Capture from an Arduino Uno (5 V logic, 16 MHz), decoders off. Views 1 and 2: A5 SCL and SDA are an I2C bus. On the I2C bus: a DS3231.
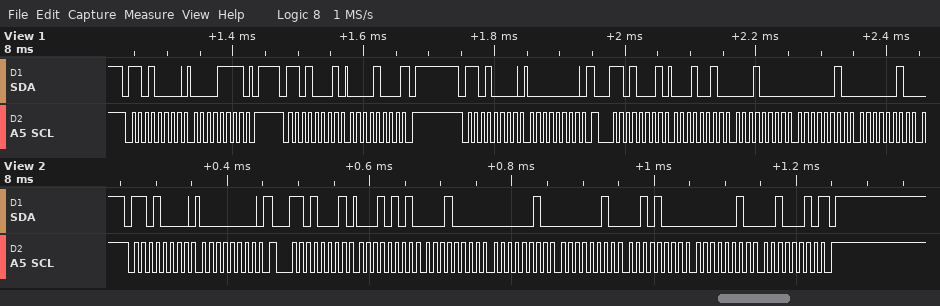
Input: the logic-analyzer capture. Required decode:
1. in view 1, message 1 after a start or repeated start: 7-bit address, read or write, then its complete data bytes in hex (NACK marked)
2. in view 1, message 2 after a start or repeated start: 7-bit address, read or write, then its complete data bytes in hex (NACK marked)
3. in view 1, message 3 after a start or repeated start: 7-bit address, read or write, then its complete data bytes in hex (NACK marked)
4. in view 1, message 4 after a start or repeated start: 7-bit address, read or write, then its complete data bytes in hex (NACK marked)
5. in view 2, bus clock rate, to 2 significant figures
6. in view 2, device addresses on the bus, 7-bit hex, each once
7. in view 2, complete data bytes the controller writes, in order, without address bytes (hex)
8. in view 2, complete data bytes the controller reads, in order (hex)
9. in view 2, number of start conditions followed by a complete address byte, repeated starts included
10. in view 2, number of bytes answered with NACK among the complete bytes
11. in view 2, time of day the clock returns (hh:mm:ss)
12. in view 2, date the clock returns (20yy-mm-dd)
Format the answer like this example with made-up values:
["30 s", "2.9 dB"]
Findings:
["0x68 write: 0F", "0x68 read: 08 NACK", "0x68 write: 00", "0x68 read: 12 10 02 02", "100 kHz", "0x68", "00", "15 10 02 02 28 02 22", "2", "1", "02:10:15", "2022-02-28"]
